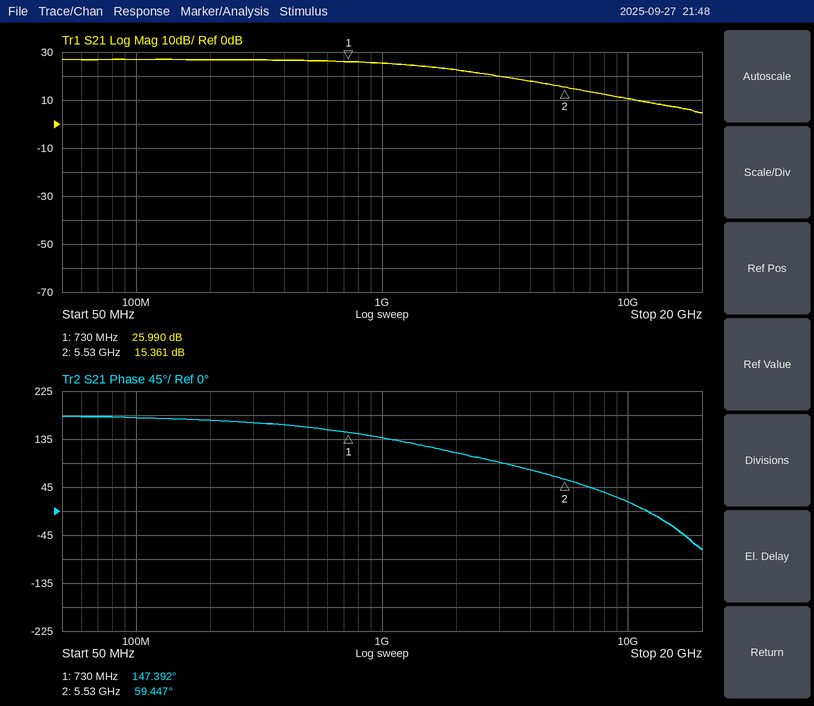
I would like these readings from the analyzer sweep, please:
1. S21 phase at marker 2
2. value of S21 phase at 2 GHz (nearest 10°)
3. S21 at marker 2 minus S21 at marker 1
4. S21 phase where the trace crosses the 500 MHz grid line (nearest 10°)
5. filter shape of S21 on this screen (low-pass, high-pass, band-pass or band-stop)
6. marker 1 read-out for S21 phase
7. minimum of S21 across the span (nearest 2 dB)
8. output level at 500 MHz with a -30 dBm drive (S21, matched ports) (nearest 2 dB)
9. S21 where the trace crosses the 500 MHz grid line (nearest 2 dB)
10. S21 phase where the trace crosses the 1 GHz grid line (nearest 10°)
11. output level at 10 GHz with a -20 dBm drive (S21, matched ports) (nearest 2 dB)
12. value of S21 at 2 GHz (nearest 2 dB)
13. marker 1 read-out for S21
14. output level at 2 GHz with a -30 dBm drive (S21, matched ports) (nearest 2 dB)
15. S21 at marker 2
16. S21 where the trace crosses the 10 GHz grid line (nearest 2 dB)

59.447°
110°
-10.629 dB
160°
low-pass
147.392°
4 dB
-4 dBm
26 dB
140°
-10 dBm
22 dB
25.990 dB
-8 dBm
15.361 dB
10 dB
